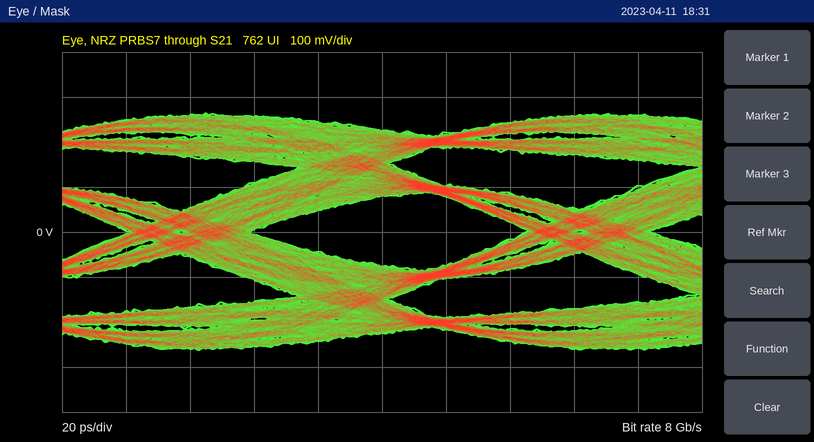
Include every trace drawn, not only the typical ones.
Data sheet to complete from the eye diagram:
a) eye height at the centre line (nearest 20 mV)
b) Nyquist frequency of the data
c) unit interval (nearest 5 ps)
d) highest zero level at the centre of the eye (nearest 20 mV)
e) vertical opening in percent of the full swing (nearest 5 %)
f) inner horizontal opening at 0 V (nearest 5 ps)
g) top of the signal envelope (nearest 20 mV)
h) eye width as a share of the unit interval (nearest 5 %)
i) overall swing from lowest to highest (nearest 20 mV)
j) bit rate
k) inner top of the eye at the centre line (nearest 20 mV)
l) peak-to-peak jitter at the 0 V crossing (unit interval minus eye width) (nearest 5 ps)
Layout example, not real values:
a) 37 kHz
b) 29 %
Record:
a) 160 mV
b) 4 GHz
c) 125 ps
d) -80 mV
e) 30 %
f) 85 ps
g) 260 mV
h) 70 %
i) 520 mV
j) 8 Gb/s
k) 80 mV
l) 40 ps
